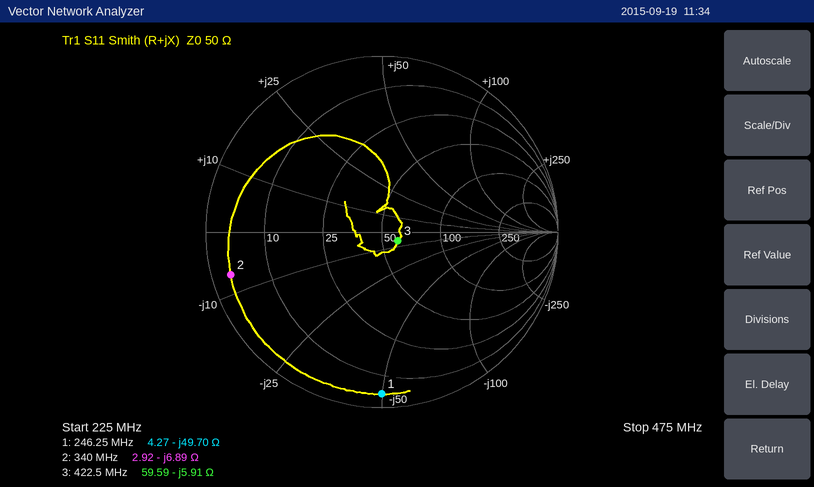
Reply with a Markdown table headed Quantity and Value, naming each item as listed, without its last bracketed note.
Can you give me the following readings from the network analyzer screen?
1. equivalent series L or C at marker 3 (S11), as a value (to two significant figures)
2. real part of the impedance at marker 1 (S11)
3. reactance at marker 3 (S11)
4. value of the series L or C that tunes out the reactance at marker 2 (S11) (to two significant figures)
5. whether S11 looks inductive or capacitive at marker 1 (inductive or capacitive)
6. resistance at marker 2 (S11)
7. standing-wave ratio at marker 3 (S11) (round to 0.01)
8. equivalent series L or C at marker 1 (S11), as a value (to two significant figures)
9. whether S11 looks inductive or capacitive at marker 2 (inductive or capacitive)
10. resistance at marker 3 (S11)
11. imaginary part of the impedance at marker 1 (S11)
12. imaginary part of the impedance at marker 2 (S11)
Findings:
| Quantity | Value |
|---|---|
| equivalent series L or C at marker 3 (S11), as a value | 64 pF |
| real part of the impedance at marker 1 | 4.27 Ω |
| reactance at marker 3 | -5.91 Ω |
| value of the series L or C that tunes out the reactance at marker 2 (S11) | 3.2 nH |
| whether S11 looks inductive or capacitive at marker 1 | capacitive |
| resistance at marker 2 | 2.92 Ω |
| standing-wave ratio at marker 3 (S11) | 1.23 |
| equivalent series L or C at marker 1 (S11), as a value | 13 pF |
| whether S11 looks inductive or capacitive at marker 2 | capacitive |
| resistance at marker 3 | 59.59 Ω |
| imaginary part of the impedance at marker 1 | -49.70 Ω |
| imaginary part of the impedance at marker 2 | -6.89 Ω |
